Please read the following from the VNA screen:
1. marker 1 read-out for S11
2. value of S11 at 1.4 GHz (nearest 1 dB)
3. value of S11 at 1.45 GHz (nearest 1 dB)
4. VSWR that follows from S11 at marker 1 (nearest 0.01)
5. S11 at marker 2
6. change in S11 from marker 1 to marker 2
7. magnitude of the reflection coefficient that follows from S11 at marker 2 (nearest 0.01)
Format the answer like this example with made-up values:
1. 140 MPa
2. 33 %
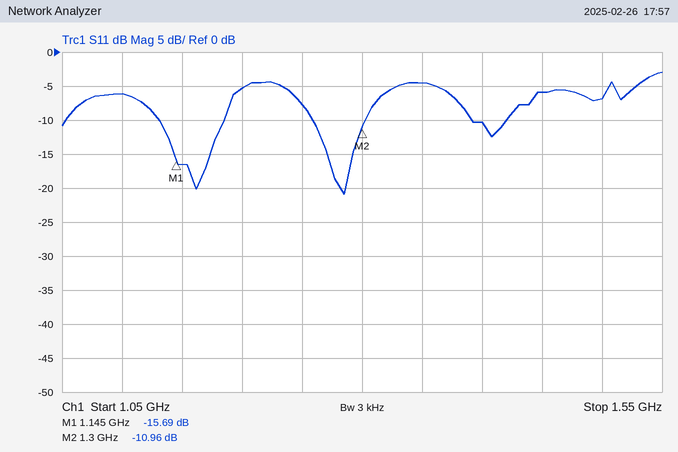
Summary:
1. -15.69 dB
2. -10 dB
3. -6 dB
4. 1.39
5. -10.96 dB
6. 4.73 dB
7. 0.28
